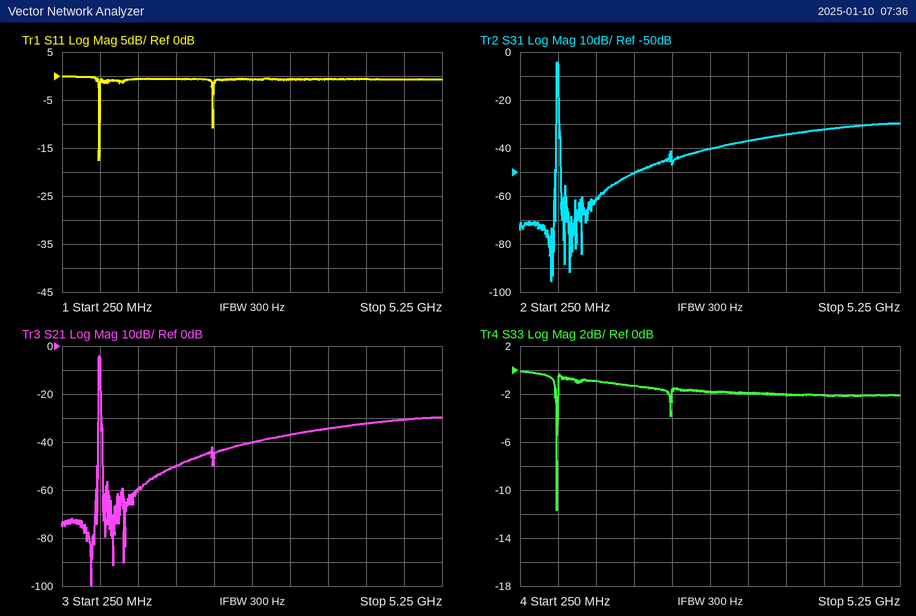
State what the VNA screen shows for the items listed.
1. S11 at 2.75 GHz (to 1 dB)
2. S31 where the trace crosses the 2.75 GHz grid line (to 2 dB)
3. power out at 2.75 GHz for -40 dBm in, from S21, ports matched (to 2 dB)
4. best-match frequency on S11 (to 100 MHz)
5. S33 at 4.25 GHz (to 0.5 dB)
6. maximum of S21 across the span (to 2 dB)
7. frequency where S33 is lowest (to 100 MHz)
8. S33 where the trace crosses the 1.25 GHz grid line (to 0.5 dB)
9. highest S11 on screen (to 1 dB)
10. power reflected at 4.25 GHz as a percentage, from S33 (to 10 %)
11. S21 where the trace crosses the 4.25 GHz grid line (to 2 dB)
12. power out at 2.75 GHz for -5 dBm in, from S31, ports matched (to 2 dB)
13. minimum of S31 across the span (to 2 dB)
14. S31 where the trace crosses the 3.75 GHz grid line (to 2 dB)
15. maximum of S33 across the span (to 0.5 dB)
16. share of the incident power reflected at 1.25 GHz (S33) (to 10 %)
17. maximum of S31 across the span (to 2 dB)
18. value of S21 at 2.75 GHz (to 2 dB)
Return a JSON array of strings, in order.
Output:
["-1 dB", "-40 dB", "-80 dBm", "700 MHz", "-2.0 dB", "-4 dB", "700 MHz", "-1.0 dB", "0 dB", "60 %", "-32 dB", "-46 dBm", "-96 dB", "-34 dB", "0.0 dB", "80 %", "-4 dB", "-40 dB"]
